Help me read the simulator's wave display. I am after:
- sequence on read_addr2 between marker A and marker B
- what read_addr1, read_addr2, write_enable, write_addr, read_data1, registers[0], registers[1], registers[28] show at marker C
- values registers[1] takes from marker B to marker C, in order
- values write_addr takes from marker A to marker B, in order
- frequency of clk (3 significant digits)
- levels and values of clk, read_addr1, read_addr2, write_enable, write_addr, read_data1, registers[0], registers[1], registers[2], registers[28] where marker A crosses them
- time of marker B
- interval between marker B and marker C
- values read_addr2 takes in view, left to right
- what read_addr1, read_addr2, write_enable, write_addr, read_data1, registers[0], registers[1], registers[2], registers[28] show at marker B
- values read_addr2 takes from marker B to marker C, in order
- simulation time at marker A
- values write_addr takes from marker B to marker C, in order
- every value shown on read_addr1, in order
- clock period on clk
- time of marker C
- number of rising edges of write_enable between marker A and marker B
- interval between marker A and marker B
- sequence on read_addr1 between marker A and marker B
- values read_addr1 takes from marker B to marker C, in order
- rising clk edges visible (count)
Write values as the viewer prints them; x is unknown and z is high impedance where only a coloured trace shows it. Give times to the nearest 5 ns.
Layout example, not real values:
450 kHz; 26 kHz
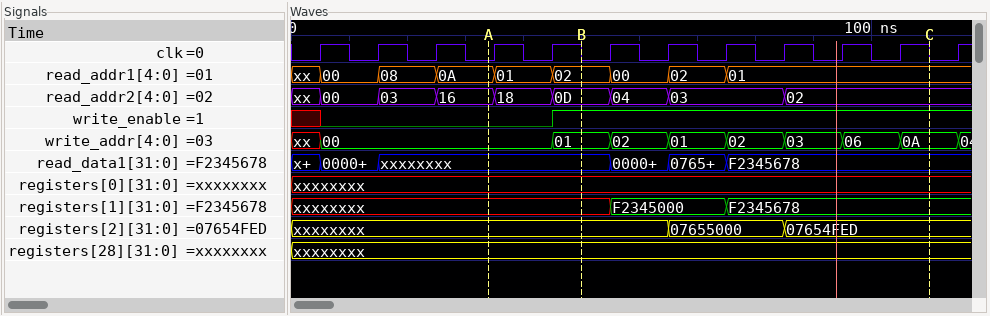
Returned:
16, 18, 0D; read_addr1=01, read_addr2=02, write_enable=1, write_addr=0A, read_data1=F2345678, registers[0]=xxxxxxxx, registers[1]=F2345678, registers[28]=xxxxxxxx; xxxxxxxx, F2345000, F2345678; 00, 01; 100 MHz; clk=0, read_addr1=0A, read_addr2=16, write_enable=0, write_addr=00, read_data1=xxxxxxxx, registers[0]=xxxxxxxx, registers[1]=xxxxxxxx, registers[2]=xxxxxxxx, registers[28]=xxxxxxxx; 50 ns; 60 ns; xx, 00, 03, 16, 18, 0D, 04, 03, 02; read_addr1=02, read_addr2=0D, write_enable=1, write_addr=01, read_data1=xxxxxxxx, registers[0]=xxxxxxxx, registers[1]=xxxxxxxx, registers[2]=xxxxxxxx, registers[28]=xxxxxxxx; 0D, 04, 03, 02; 35 ns; 01, 02, 01, 02, 03, 06, 0A; xx, 00, 08, 0A, 01, 02, 00, 02, 01; 10 ns; 110 ns; 1; 15 ns; 0A, 01, 02; 02, 00, 02, 01; 12
